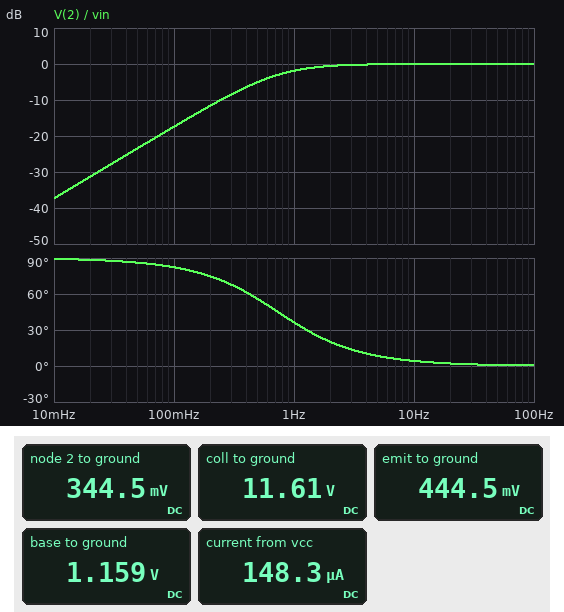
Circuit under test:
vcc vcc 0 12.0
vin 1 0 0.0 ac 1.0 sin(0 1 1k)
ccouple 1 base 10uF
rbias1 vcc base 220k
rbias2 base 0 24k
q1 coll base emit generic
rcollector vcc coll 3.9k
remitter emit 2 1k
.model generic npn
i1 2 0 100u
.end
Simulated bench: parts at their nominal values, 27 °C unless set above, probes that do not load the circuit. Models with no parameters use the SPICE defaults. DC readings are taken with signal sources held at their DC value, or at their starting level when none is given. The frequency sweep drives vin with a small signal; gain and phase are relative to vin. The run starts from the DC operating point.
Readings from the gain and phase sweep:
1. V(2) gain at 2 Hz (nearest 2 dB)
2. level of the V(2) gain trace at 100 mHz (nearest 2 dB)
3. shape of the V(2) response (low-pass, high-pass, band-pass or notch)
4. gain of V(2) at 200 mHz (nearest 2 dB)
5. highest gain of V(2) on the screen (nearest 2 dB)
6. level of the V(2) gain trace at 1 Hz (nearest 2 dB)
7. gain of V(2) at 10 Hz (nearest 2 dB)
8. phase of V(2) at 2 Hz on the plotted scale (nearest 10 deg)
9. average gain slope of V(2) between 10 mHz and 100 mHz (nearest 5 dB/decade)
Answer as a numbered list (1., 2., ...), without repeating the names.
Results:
1. 0 dB
2. -18 dB
3. high-pass
4. -12 dB
5. 0 dB
6. -2 dB
7. 0 dB
8. 20 deg
9. 20 dB/decade
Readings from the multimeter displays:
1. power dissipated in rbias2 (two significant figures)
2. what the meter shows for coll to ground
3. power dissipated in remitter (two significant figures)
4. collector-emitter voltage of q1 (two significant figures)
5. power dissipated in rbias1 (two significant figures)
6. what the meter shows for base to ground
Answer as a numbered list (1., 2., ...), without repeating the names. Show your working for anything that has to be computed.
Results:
1. (1.159 V)^2 / 24 kΩ = 56 µW
2. 11.61 V
3. (444.5 mV - 344.5 mV)^2 / 1 kΩ = 10 µW
4. 11.61 V - 444.5 mV = 11 V
5. (12 V - 1.159 V)^2 / 220 kΩ = 530 µW
6. 1.159 V
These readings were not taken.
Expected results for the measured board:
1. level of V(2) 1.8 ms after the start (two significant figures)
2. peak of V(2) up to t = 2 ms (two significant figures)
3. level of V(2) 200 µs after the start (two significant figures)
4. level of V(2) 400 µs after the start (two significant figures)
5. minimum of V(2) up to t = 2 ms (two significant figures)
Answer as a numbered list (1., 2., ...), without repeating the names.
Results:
1. -610 mV
2. 1.3 V
3. 1.3 V
4. 930 mV
5. -660 mV
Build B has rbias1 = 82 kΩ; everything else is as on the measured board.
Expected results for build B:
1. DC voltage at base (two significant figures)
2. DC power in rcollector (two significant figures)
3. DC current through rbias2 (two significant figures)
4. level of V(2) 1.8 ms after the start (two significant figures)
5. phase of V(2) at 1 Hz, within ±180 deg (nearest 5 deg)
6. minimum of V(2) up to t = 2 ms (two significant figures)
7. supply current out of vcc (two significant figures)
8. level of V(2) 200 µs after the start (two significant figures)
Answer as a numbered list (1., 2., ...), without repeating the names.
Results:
1. 2.7 V
2. 38 µW
3. 110 µA
4. 930 mV
5. 40 deg
6. 880 mV
7. 210 µA
8. 2.8 V
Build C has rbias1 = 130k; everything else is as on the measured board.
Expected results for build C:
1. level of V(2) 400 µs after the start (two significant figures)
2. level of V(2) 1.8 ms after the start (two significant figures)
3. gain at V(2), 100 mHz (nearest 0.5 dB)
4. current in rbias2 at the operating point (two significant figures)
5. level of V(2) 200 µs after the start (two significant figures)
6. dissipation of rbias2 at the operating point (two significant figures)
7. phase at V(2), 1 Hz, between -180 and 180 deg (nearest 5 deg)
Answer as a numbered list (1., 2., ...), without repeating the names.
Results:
1. 1.6 V
2. 84 mV
3. -18.0 dB
4. 77 µA
5. 2.0 V
6. 140 µW
7. 40 deg
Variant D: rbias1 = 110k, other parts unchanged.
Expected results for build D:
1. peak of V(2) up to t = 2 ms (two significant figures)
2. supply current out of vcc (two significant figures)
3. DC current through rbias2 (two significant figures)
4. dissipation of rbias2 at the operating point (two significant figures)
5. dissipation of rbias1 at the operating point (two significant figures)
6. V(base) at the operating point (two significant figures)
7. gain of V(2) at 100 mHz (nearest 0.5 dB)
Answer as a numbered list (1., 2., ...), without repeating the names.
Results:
1. 2.3 V
2. 190 µA
3. 89 µA
4. 190 µW
5. 890 µW
6. 2.1 V
7. -18.0 dB
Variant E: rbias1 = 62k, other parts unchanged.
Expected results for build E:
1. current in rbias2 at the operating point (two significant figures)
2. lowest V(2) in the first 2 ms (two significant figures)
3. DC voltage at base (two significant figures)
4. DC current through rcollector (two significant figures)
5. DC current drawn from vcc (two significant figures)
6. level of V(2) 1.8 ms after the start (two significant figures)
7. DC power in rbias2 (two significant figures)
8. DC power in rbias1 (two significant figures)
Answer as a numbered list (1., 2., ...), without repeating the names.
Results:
1. 140 µA
2. 1.5 V
3. 3.3 V
4. 99 µA
5. 240 µA
6. 1.6 V
7. 460 µW
8. 1.2 mW
